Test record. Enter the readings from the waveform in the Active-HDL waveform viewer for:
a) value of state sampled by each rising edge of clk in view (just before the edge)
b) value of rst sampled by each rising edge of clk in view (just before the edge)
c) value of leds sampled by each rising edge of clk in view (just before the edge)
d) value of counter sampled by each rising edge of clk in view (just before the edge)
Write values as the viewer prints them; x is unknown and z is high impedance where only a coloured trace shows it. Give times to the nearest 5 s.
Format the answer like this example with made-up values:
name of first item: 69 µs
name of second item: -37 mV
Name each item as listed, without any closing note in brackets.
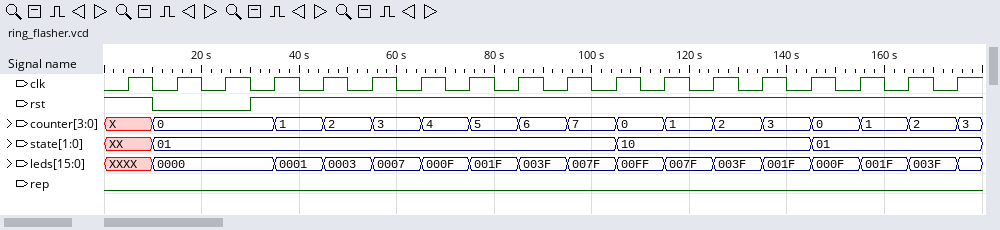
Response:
value of state sampled by each rising edge of clk in view: XX, 01, 01, 01, 01, 01, 01, 01, 01, 01, 01, 10, 10, 10, 10, 01, 01, 01
value of rst sampled by each rising edge of clk in view: 1 0 0 1 1 1 1 1 1 1 1 1 1 1 1 1 1 1
value of leds sampled by each rising edge of clk in view: XXXX, 0000, 0000, 0000, 0001, 0003, 0007, 000F, 001F, 003F, 007F, 00FF, 007F, 003F, 001F, 000F, 001F, 003F
value of counter sampled by each rising edge of clk in view: X, 0, 0, 0, 1, 2, 3, 4, 5, 6, 7, 0, 1, 2, 3, 0, 1, 2
